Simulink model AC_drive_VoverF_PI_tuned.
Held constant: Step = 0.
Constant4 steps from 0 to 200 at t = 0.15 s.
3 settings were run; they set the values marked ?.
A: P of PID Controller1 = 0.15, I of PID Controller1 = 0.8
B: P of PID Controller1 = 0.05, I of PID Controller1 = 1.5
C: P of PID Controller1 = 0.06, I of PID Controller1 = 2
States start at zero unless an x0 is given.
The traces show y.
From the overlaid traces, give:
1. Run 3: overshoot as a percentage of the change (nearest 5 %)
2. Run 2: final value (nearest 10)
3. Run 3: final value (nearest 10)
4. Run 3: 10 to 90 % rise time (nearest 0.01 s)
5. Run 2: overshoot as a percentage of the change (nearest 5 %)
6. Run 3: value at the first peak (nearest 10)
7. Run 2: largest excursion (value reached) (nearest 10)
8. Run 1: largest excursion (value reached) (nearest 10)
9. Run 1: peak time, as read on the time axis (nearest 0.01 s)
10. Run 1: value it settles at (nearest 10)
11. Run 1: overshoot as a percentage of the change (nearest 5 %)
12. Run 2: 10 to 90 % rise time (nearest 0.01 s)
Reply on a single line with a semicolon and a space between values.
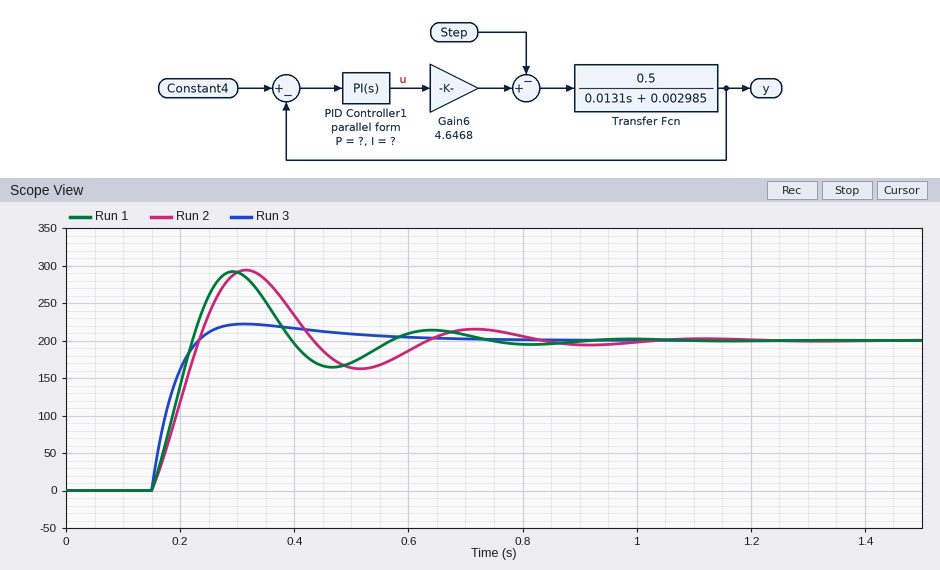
10 %; 200; 200; 0.06 s; 45 %; 220; 290; 290; 0.29 s; 200; 45 %; 0.06 s
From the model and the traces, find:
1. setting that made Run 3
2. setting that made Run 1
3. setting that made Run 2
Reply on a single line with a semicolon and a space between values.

A; C; B
